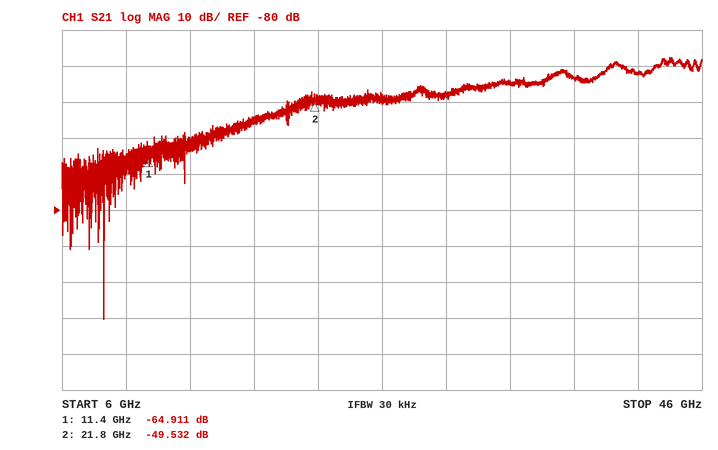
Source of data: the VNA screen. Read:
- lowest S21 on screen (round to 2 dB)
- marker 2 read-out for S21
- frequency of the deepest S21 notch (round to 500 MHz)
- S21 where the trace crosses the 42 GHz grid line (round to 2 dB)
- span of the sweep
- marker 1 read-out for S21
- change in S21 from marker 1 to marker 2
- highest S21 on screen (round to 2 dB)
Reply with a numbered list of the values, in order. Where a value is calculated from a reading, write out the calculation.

1. -110 dB
2. -49.532 dB
3. 8.5 GHz
4. -42 dB
5. 40 GHz
6. -64.911 dB
7. -49.532 − (-64.911) = 15.379 dB
8. -38 dB
